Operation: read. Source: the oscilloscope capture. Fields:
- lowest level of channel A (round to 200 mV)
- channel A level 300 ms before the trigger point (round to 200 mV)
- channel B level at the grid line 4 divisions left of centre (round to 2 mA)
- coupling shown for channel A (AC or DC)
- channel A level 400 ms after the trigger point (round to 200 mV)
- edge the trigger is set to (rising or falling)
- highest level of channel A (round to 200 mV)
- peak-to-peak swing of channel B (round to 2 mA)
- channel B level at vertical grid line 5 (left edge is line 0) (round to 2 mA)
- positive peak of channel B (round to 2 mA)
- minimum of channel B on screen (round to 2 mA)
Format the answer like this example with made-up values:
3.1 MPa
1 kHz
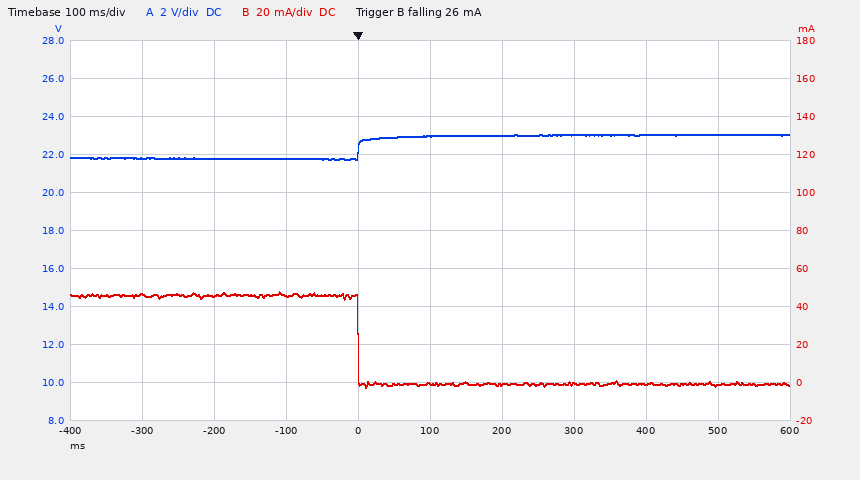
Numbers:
21.8 V
21.8 V
46 mA
DC
23.0 V
falling
23.0 V
50 mA
0 mA
48 mA
-2 mA
